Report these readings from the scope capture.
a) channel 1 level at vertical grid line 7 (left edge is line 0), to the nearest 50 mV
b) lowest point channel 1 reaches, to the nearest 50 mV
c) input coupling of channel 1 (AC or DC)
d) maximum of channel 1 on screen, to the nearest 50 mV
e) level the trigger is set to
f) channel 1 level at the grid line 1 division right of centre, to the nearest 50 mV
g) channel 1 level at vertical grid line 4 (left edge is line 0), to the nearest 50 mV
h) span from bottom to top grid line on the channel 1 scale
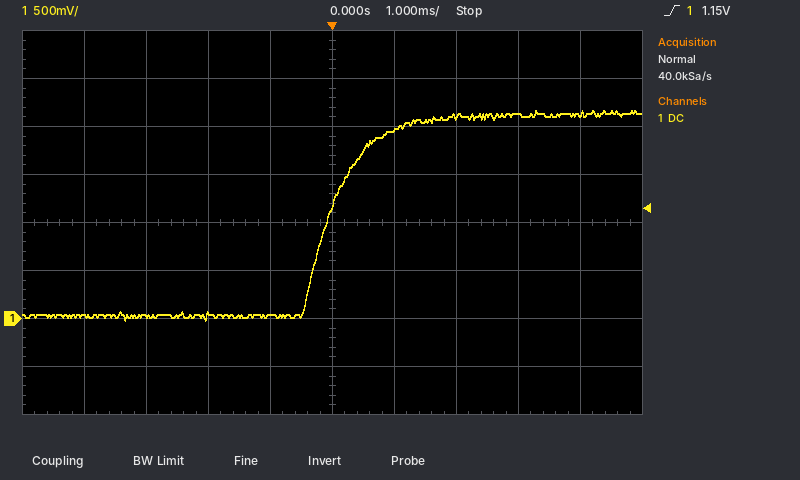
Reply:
2.10 V
0 mV
DC
2.15 V
1.15 V
1.95 V
50 mV
4 V
